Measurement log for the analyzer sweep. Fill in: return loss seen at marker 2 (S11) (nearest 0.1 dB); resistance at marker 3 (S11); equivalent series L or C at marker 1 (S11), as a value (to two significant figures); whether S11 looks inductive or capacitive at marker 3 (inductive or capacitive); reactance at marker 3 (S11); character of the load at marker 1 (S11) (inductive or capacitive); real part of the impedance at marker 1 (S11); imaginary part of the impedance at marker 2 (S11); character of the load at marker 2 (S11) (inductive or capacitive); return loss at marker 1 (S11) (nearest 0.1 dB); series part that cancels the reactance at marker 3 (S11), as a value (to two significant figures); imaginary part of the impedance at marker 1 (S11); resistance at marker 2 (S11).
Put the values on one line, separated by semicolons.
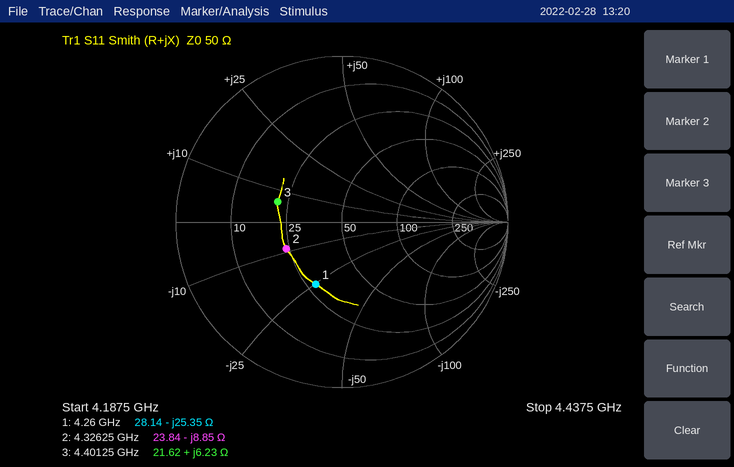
8.6 dB; 21.62 Ω; 1.5 pF; inductive; +6.23 Ω; capacitive; 28.14 Ω; -8.85 Ω; capacitive; 7.8 dB; 5.8 pF; -25.35 Ω; 23.84 Ω
